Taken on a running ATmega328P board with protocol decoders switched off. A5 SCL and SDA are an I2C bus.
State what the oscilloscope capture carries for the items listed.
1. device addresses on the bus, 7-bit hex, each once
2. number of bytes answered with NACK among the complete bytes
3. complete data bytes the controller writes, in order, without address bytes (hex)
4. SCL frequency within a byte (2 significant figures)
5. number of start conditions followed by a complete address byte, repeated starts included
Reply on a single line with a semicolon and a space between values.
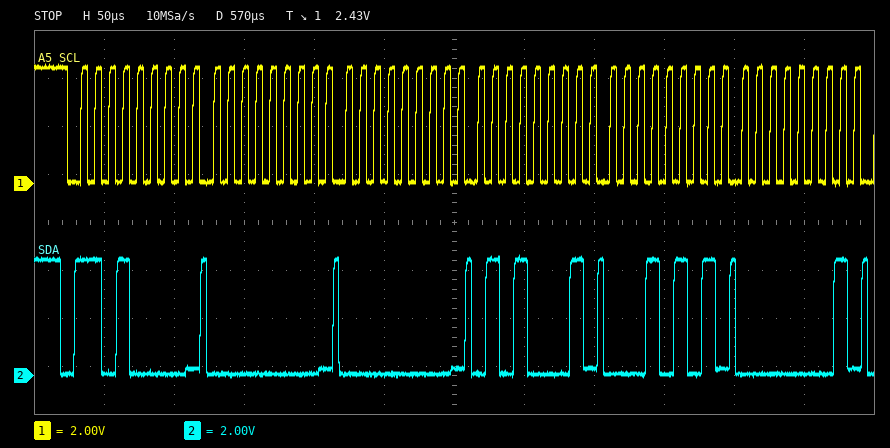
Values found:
0x68; 0; 00 00 51 15 01; 100 kHz; 1
